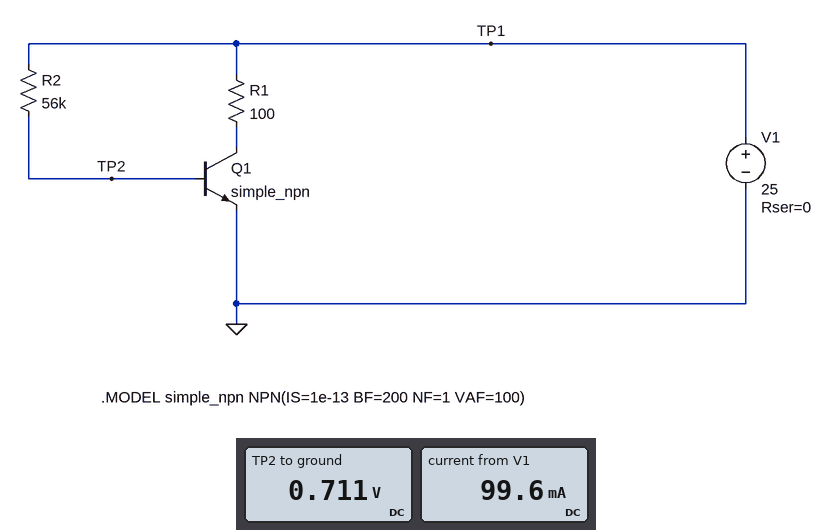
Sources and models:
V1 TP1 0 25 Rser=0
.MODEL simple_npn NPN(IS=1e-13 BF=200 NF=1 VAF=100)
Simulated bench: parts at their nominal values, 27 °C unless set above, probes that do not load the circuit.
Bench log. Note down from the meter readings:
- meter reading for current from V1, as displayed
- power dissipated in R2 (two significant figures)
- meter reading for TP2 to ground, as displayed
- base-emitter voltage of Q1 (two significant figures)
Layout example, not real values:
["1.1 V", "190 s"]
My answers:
["99.6 mA", "11 mW", "0.711 V", "710 mV"]
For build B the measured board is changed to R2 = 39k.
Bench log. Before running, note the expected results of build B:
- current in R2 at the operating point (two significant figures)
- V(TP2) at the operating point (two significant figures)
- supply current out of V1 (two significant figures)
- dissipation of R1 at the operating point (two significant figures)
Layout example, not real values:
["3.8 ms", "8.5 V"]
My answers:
["620 µA", "720 mV", "140 mA", "1.9 W"]
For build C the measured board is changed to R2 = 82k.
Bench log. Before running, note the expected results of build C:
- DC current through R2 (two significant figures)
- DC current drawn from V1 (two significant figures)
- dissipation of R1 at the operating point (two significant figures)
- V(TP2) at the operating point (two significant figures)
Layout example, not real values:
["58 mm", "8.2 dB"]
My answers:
["300 µA", "70 mA", "480 mW", "700 mV"]
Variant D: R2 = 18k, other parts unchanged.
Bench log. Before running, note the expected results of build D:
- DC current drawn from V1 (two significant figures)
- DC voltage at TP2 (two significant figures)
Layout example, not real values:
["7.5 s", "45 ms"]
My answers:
["250 mA", "740 mV"]
